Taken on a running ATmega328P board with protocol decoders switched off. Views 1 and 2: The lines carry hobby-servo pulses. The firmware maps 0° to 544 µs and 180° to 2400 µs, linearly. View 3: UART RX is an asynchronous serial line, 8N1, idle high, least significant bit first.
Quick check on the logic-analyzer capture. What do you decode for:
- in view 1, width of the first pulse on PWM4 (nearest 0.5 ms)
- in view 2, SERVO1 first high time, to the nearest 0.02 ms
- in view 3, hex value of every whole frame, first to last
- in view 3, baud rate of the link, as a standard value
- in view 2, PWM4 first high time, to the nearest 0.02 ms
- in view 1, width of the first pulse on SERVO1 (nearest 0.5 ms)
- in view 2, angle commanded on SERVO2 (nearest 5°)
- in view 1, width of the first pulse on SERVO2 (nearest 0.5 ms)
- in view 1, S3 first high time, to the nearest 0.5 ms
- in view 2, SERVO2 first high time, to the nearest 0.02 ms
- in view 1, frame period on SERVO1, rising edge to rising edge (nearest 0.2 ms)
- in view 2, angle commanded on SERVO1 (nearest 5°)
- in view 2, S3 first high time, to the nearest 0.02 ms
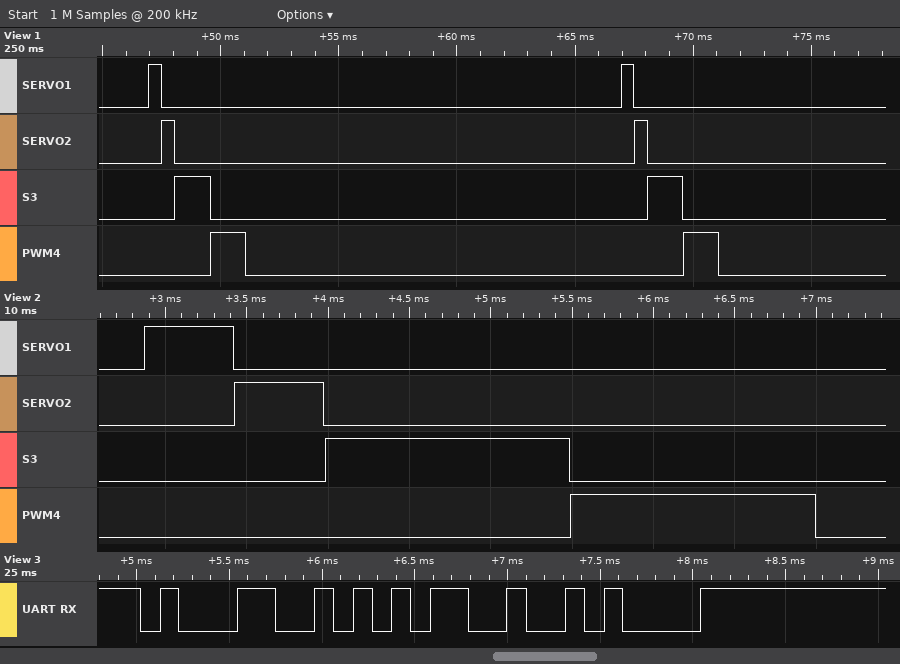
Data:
1.5 ms
0.54 ms
31 35 0A
9600 baud
1.50 ms
0.5 ms
0°
0.5 ms
1.5 ms
0.54 ms
20.0 ms
0°
1.50 ms
